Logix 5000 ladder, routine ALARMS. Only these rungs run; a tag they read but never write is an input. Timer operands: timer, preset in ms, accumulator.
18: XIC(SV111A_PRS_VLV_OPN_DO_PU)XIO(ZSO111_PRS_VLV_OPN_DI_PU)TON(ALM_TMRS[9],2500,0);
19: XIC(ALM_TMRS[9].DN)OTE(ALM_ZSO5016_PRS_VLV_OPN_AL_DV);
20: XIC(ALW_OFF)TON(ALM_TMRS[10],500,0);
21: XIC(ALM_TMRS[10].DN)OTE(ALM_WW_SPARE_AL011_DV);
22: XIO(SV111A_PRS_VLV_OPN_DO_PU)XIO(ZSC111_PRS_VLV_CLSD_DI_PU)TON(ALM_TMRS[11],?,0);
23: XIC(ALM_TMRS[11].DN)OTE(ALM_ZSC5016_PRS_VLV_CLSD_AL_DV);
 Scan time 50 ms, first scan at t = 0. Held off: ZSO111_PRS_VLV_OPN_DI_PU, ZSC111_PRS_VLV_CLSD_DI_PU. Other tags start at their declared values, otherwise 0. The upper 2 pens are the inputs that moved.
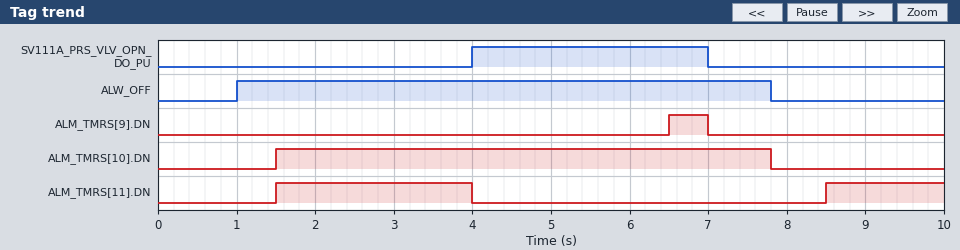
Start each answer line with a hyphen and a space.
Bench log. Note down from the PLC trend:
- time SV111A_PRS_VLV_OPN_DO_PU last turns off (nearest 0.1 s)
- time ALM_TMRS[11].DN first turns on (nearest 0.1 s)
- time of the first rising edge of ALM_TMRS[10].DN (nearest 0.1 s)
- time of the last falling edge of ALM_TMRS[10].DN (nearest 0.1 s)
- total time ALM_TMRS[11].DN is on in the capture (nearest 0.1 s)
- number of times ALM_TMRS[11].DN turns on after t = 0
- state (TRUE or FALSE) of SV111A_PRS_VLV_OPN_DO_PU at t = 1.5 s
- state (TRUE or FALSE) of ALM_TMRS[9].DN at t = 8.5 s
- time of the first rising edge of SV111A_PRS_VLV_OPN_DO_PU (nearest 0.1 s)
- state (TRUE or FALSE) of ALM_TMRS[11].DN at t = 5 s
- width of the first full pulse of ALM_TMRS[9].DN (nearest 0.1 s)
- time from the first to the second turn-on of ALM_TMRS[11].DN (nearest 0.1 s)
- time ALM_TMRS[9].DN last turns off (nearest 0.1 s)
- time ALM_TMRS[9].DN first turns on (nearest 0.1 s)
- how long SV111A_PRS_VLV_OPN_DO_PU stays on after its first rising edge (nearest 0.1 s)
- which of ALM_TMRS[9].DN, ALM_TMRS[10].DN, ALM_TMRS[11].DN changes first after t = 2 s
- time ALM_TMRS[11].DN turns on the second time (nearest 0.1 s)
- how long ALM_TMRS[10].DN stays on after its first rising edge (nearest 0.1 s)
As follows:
- 7.0 s
- 1.5 s
- 1.5 s
- 7.8 s
- 4.0 s
- 2
- FALSE
- FALSE
- 4.0 s
- FALSE
- 0.5 s
- 7.0 s
- 7.0 s
- 6.5 s
- 3.0 s
- ALM_TMRS[11].DN
- 8.5 s
- 6.3 s
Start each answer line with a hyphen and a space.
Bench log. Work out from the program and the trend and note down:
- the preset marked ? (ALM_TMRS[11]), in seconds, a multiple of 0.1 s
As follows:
- 1.5 s
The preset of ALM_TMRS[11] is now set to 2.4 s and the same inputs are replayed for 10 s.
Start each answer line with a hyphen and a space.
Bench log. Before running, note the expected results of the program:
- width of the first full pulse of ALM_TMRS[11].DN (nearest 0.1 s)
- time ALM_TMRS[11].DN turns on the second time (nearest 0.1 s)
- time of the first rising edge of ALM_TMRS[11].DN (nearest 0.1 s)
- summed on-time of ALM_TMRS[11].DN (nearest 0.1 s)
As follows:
- 1.6 s
- 9.4 s
- 2.4 s
- 2.2 s
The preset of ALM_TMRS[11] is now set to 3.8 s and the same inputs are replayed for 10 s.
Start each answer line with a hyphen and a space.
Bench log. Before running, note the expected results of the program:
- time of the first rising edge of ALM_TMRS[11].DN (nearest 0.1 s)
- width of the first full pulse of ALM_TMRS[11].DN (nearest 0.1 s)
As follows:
- 3.8 s
- 0.2 s
